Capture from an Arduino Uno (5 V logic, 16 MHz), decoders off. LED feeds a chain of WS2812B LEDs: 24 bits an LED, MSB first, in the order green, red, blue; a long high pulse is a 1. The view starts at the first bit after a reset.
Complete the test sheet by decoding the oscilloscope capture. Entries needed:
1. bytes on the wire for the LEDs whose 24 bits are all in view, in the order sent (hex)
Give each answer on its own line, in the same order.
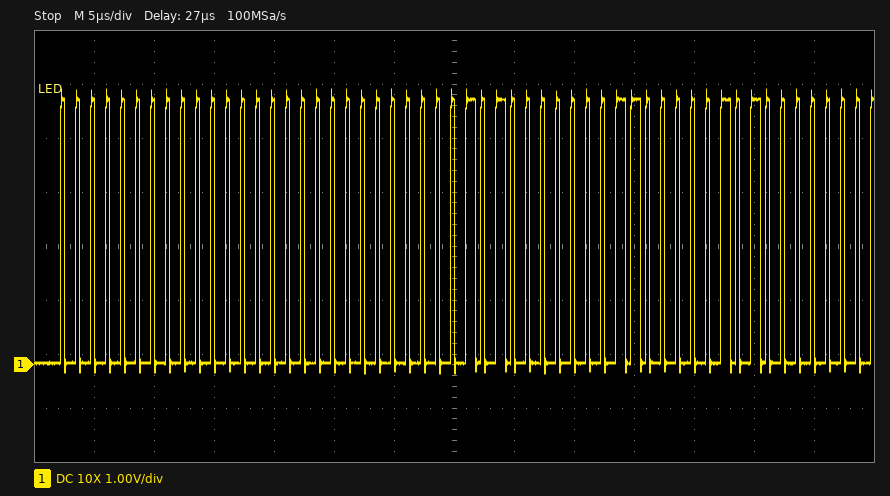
00 00 00 14 06 0A
